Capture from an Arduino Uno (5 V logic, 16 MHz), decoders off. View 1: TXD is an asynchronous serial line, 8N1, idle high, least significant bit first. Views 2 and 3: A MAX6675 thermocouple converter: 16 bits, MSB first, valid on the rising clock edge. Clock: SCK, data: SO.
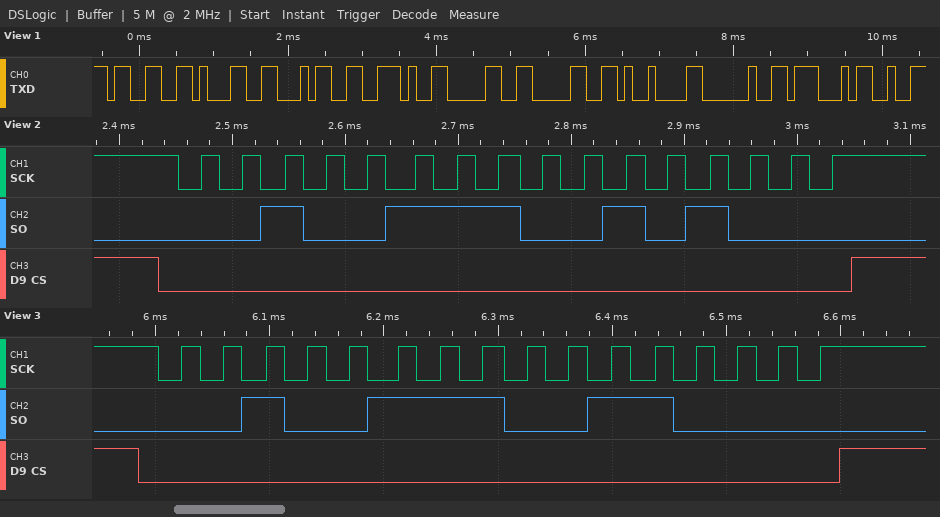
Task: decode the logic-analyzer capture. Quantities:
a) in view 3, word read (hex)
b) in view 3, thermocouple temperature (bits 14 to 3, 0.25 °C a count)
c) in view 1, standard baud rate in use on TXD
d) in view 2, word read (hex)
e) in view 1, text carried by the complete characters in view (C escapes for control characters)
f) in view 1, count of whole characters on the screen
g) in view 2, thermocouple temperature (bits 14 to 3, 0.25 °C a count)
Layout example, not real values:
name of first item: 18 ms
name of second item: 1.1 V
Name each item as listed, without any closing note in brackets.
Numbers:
in view 3, word read: 0x2730
in view 3, thermocouple temperature: 313.50 °C
in view 1, standard baud rate in use on TXD: 9600 baud
in view 2, word read: 0x2728
in view 1, text carried by the complete characters in view: "314.00\t G"
in view 1, count of whole characters on the screen: 9
in view 2, thermocouple temperature: 313.25 °C
